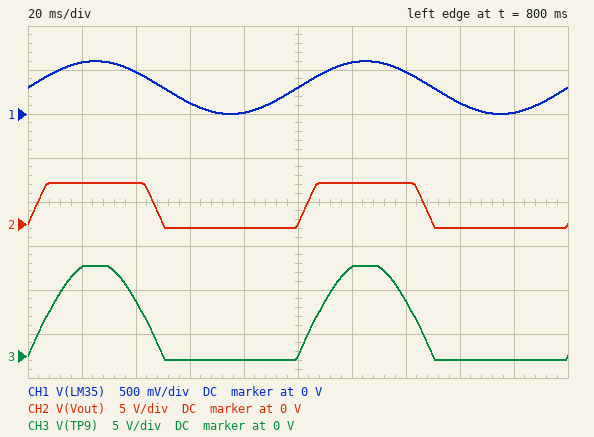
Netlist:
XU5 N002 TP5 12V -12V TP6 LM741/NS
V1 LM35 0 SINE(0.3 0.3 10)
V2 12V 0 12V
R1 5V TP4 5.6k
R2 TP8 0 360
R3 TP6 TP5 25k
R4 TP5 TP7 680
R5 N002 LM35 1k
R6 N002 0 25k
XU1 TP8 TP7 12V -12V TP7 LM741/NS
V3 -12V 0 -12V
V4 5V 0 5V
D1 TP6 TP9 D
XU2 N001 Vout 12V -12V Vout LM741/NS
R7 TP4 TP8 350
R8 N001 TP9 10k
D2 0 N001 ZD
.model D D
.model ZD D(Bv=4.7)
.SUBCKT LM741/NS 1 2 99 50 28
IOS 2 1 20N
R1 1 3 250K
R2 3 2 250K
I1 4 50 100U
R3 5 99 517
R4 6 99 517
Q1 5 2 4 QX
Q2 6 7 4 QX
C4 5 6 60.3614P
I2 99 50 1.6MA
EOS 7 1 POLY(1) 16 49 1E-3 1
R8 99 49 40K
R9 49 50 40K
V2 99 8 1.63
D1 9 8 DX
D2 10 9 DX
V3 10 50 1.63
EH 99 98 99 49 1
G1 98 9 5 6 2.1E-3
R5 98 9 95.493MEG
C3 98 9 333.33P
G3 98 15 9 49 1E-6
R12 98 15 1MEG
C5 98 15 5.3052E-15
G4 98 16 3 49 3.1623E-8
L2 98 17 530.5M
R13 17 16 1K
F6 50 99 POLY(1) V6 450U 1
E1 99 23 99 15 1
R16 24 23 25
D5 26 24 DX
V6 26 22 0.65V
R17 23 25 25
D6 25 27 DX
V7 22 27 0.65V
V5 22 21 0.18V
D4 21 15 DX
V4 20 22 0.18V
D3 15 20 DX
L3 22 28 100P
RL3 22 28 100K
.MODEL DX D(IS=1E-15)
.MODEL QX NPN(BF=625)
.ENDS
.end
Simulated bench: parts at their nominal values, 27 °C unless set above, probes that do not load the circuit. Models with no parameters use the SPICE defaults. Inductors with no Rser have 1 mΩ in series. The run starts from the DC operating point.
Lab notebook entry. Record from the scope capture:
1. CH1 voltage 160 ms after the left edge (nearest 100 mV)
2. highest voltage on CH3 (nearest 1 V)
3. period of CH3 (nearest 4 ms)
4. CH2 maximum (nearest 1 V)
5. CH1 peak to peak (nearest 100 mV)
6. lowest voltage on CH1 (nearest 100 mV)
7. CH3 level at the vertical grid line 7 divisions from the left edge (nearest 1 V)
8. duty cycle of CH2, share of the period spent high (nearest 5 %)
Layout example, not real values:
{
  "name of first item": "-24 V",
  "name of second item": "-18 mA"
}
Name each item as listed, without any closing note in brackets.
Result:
{
  "CH1 voltage 160 ms after the left edge": "100 mV",
  "highest voltage on CH3": "10 V",
  "period of CH3": "100 ms",
  "CH2 maximum": "5 V",
  "CH1 peak to peak": "600 mV",
  "lowest voltage on CH1": "0 V",
  "CH3 level at the vertical grid line 7 divisions from the left edge": "6 V",
  "duty cycle of CH2, share of the period spent high": "45 %"
}
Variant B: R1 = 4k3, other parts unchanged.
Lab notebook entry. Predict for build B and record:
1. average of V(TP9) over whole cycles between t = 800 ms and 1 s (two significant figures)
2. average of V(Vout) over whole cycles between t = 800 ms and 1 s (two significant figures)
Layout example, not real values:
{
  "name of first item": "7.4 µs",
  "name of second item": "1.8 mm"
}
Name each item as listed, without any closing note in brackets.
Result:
{
  "average of V(TP9) over whole cycles between t = 800 ms and 1 s": "1.9 V",
  "average of V(Vout) over whole cycles between t = 800 ms and 1 s": "1.4 V"
}
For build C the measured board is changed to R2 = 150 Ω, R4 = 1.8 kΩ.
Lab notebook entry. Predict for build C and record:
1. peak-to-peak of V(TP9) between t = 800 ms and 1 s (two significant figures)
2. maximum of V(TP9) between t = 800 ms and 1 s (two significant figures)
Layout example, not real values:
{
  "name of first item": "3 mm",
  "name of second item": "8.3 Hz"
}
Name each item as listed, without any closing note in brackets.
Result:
{
  "peak-to-peak of V(TP9) between t = 800 ms and 1 s": "6.7 V",
  "maximum of V(TP9) between t = 800 ms and 1 s": "6.3 V"
}
